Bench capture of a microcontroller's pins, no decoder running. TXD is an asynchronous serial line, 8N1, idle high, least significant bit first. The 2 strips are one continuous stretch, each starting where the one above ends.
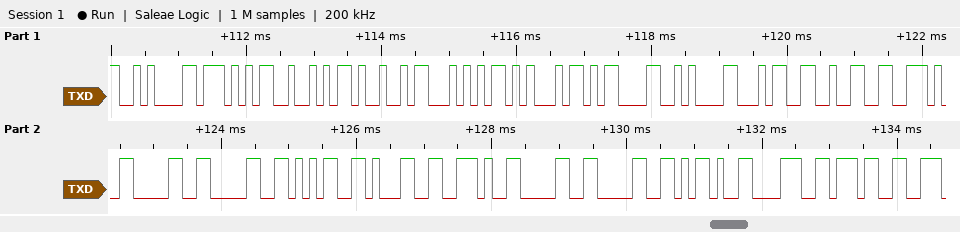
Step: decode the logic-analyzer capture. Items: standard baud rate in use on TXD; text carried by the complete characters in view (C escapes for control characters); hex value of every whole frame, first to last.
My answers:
9600 baud
"\nWRITE\r\n42.0051.00-87"
0A 57 52 49 54 45 0D 0A 34 32 2E 30 30 35 31 2E 30 30 2D 38 37
